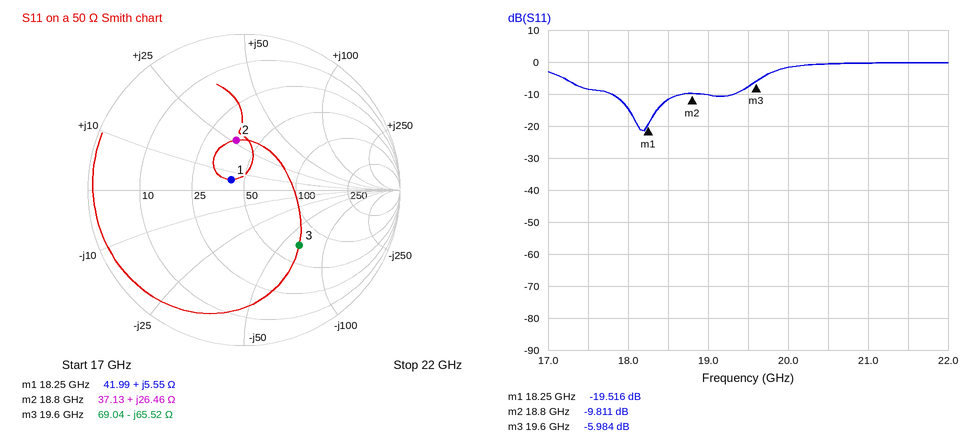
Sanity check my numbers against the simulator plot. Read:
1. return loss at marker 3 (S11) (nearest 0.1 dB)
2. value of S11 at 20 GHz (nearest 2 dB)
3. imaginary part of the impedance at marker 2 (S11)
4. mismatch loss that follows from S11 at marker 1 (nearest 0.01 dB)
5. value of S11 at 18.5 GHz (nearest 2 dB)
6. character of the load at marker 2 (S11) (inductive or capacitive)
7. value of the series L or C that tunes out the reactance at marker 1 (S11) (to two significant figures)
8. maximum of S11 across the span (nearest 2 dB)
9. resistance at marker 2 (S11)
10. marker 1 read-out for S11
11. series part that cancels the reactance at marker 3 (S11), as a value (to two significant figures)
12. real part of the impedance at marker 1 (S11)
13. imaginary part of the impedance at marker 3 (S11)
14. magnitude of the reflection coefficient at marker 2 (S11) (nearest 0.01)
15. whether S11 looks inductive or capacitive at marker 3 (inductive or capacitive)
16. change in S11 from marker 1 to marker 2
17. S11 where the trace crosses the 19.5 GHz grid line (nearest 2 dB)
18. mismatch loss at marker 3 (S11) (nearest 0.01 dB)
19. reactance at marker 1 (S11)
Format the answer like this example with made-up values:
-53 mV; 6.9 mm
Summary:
6.0 dB; -2 dB; +26.46 Ω; 0.05 dB; -12 dB; inductive; 1.6 pF; 0 dB; 37.13 Ω; -19.516 dB; 530 pH; 41.99 Ω; -65.52 Ω; 0.32; capacitive; 9.705 dB; -8 dB; 1.26 dB; +5.55 Ω
